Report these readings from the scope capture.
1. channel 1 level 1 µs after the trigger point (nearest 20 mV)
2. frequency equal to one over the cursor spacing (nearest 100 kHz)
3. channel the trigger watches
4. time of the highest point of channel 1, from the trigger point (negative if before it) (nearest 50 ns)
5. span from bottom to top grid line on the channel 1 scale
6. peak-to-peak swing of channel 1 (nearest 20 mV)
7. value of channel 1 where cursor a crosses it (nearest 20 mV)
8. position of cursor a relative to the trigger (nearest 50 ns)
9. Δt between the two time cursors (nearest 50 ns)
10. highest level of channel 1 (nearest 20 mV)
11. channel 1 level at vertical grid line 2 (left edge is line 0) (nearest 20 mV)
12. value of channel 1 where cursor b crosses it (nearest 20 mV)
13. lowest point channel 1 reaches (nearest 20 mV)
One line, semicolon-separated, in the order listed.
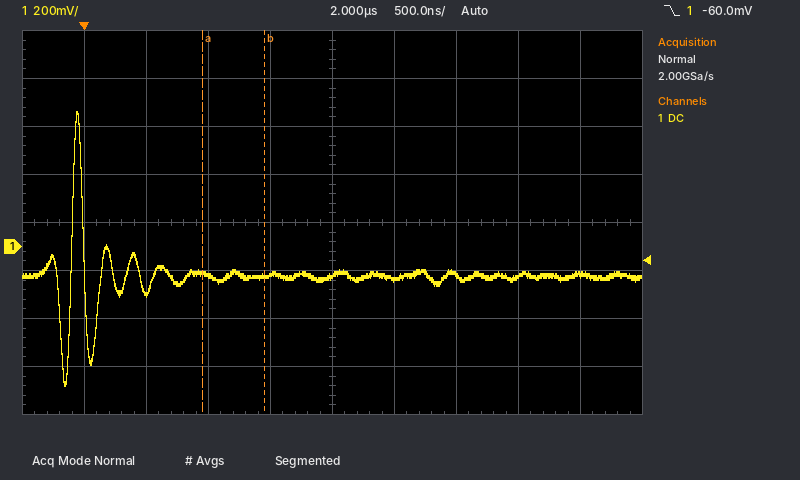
-120 mV; 2.0 MHz; channel 1; -50 ns; 1.6 V; 1.14 V; -120 mV; +950 ns; 500 ns; 560 mV; -200 mV; -120 mV; -580 mV
